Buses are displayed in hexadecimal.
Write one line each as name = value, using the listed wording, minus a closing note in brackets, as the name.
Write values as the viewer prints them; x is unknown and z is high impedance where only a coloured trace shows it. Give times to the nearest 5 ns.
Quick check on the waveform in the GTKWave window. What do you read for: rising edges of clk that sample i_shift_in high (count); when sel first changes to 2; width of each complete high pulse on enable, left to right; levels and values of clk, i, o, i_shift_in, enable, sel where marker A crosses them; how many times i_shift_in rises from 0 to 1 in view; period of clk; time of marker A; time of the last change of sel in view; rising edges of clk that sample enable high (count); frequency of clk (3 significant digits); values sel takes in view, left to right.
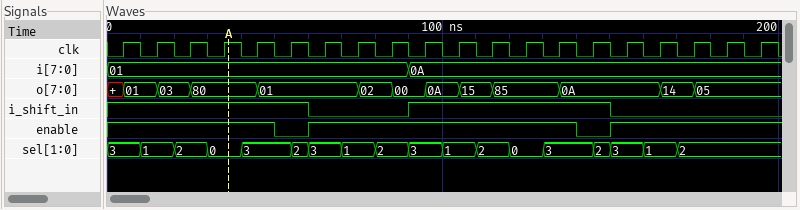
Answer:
rising edges of clk that sample i_shift_in high = 12
when sel first changes to 2 = 20 ns
width of each complete high pulse on enable, left to right = 80 ns
levels and values of clk, i, o, i_shift_in, enable, sel where marker A crosses them = clk=1, i=01, o=80, i_shift_in=1, enable=1, sel=0
how many times i_shift_in rises from 0 to 1 in view = 1
period of clk = 10 ns
time of marker A = 35 ns
time of the last change of sel in view = 170 ns
rising edges of clk that sample enable high = 18
frequency of clk = 100 MHz
values sel takes in view, left to right = 3, 1, 2, 0, 3, 2, 3, 1, 2, 3, 1, 2, 0, 3, 2, 3, 1, 2
